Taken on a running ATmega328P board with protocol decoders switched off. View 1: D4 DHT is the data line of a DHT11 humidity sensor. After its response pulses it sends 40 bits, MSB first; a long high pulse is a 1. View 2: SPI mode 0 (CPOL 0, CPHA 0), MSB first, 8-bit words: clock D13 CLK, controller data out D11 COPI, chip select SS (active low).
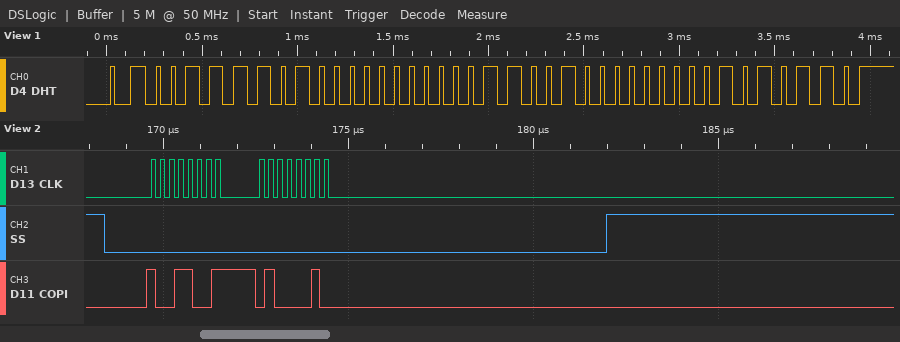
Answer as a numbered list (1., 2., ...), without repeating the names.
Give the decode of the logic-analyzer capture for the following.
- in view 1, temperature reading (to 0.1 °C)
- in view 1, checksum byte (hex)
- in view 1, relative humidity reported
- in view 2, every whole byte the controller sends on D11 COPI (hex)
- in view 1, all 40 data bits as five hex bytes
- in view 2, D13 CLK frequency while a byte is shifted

1. 25.0 °C
2. 0x56
3. 61 %
4. 0x99 0x42
5. 3D 00 19 00 56
6. 4 MHz
